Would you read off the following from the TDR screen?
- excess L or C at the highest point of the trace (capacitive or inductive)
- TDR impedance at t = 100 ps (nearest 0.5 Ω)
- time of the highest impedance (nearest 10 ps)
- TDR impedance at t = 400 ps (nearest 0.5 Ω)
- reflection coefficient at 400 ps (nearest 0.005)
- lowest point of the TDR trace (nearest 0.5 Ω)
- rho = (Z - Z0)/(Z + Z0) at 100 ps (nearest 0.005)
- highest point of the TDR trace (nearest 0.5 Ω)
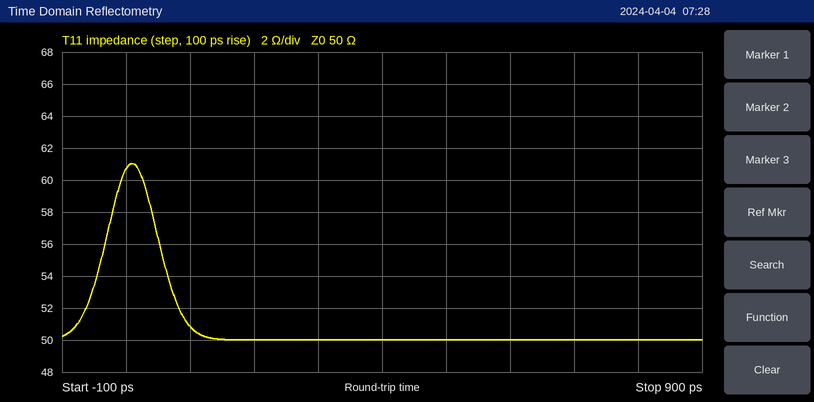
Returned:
inductive
51.0 Ω
10 ps
50.0 Ω
0.000
50.0 Ω
+0.010
61.0 Ω
